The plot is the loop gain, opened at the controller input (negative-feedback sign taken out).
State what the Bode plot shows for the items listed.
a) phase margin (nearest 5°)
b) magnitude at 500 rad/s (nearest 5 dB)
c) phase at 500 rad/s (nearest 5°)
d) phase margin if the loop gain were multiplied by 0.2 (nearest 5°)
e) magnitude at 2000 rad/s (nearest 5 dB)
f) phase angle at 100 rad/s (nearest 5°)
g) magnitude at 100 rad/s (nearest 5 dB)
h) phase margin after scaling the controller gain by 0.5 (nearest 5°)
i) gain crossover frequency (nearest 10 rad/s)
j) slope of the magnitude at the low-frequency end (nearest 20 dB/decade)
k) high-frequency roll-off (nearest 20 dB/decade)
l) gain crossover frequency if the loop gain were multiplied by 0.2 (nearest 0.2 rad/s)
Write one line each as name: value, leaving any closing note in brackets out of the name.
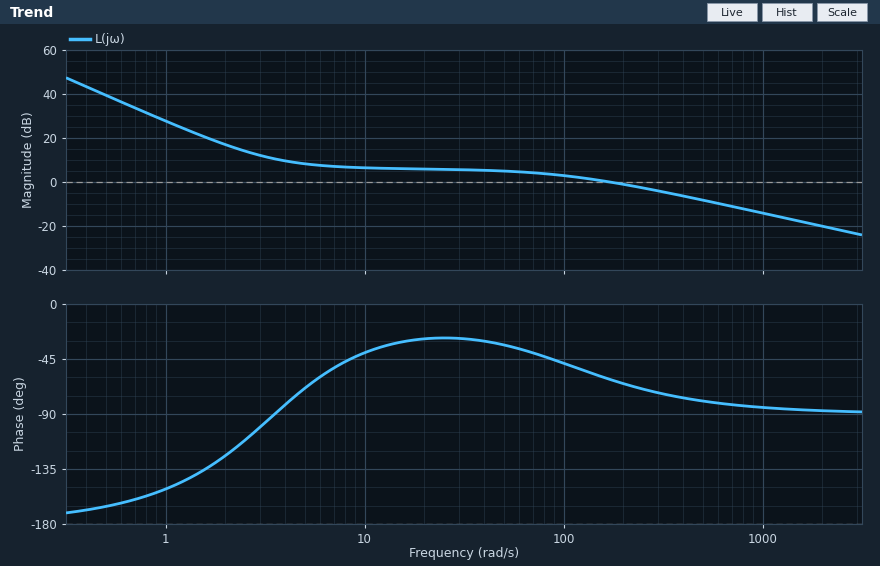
phase margin: 120°
magnitude at 500 rad/s: -10 dB
phase at 500 rad/s: -80°
phase margin if the loop gain were multiplied by 0.2: 70°
magnitude at 2000 rad/s: -20 dB
phase angle at 100 rad/s: -50°
magnitude at 100 rad/s: 5 dB
phase margin after scaling the controller gain by 0.5: 150°
gain crossover frequency: 170 rad/s
slope of the magnitude at the low-frequency end: -40 dB/decade
high-frequency roll-off: -20 dB/decade
gain crossover frequency if the loop gain were multiplied by 0.2: 2.6 rad/s
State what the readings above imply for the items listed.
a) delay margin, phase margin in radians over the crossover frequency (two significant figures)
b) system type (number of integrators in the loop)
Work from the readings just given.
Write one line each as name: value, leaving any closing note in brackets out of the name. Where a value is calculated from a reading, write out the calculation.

delay margin, phase margin in radians over the crossover frequency: 120 × π / 180 / 170 = 0.012 s
system type: 2
